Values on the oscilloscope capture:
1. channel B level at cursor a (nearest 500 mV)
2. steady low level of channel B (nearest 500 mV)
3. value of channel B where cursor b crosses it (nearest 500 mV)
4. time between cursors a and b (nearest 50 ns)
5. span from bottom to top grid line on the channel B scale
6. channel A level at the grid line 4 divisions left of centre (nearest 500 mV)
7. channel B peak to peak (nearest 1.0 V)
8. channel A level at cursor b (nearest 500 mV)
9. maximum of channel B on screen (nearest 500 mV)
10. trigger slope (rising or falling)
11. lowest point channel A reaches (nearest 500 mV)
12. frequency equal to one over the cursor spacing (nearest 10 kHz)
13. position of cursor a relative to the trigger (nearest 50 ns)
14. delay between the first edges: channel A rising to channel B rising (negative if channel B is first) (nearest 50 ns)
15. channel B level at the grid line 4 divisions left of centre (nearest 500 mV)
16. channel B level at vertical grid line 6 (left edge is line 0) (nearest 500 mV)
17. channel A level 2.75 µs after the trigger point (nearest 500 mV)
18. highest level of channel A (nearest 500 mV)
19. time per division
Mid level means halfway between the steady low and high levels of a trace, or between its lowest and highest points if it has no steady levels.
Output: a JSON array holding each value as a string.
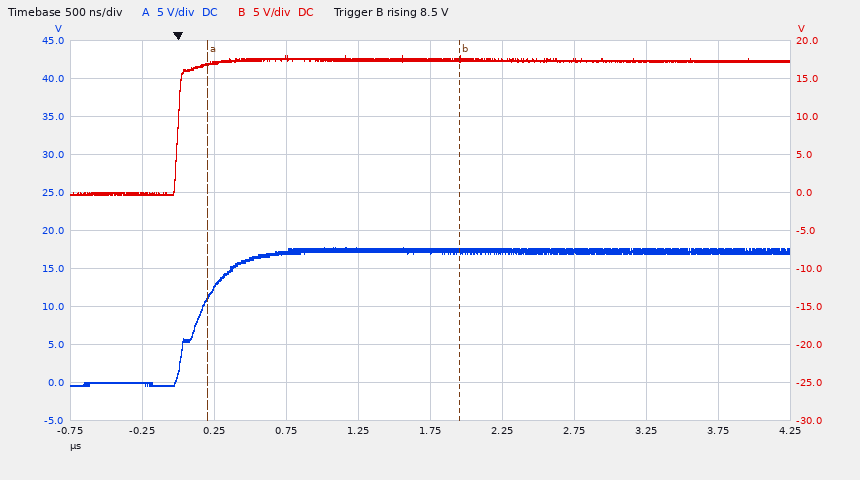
["17.0 V", "0.0 V", "17.5 V", "1.75 µs", "50 V", "0.0 V", "18.0 V", "17.5 V", "18.0 V", "rising", "-500 mV", "570 kHz", "+200 ns", "-150 ns", "0.0 V", "17.5 V", "17.5 V", "18.0 V", "500 ns"]
